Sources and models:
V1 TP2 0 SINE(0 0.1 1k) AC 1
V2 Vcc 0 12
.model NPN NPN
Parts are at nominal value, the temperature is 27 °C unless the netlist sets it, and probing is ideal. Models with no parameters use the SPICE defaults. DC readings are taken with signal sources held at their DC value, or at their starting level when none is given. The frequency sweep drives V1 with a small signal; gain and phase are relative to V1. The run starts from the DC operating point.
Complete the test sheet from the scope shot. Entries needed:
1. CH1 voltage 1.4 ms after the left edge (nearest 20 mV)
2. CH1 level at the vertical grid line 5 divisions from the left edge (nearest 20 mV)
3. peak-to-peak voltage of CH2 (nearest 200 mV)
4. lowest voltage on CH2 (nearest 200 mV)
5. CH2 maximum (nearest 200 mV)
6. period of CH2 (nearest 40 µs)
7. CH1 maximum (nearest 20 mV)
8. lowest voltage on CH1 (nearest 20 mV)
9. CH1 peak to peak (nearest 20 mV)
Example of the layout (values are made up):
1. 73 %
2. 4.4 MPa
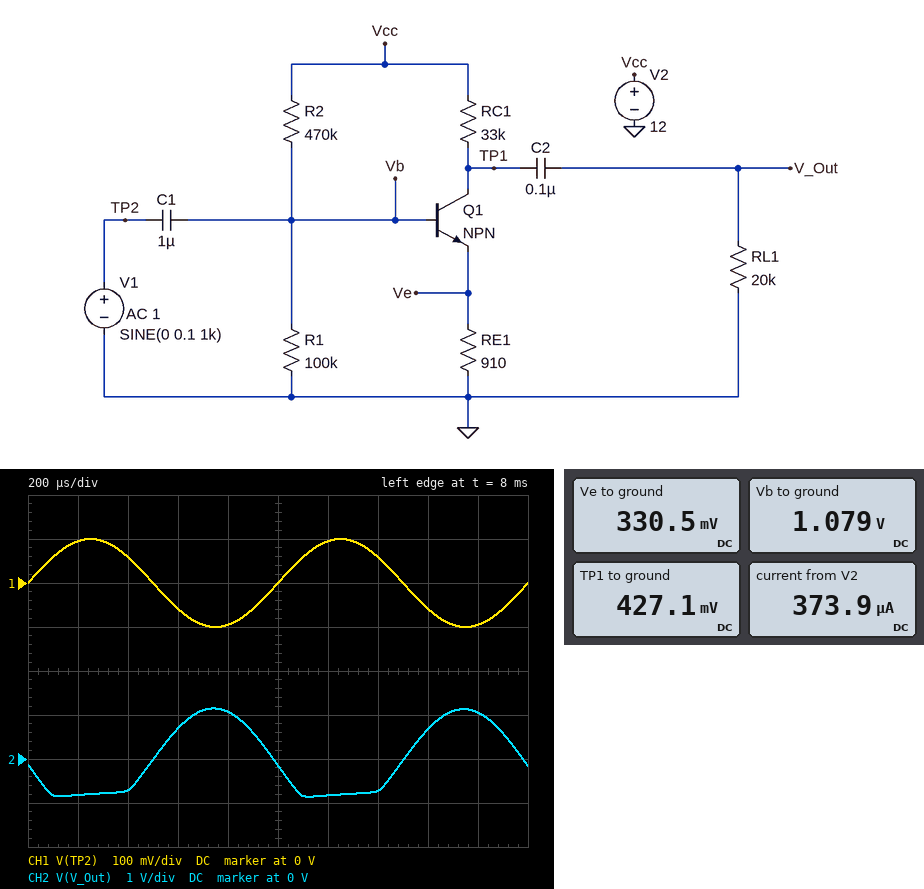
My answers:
1. 60 mV
2. 0 V
3. 2.0 V
4. -800 mV
5. 1.2 V
6. 1.00 ms
7. 100 mV
8. -100 mV
9. 200 mV
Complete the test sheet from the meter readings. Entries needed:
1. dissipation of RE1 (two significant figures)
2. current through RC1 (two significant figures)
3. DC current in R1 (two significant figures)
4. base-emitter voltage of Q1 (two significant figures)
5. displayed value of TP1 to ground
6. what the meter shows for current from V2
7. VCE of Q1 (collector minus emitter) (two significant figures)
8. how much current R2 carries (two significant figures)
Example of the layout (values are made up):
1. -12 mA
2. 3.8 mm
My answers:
1. 120 µW
2. 350 µA
3. 11 µA
4. 750 mV
5. 427.1 mV
6. 373.9 µA
7. 97 mV
8. 23 µA
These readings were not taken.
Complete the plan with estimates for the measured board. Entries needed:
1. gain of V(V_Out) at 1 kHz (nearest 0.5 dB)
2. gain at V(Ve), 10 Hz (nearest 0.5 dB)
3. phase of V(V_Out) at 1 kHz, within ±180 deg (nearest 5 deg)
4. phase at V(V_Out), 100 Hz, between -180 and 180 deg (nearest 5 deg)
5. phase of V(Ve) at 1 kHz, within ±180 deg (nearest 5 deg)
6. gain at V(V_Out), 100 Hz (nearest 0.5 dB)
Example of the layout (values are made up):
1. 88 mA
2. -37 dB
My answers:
1. 3.0 dB
2. -24.5 dB
3. -170 deg
4. -90 deg
5. 10 deg
6. -3.0 dB
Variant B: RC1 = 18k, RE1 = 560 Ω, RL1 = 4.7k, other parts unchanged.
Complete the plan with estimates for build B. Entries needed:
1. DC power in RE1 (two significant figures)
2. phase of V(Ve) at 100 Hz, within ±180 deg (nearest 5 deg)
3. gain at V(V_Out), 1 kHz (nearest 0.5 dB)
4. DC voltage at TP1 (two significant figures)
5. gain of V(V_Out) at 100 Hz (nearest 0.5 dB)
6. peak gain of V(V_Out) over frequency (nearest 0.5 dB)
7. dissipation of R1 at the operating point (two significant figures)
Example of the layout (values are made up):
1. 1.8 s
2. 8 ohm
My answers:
1. 240 µW
2. 70 deg
3. 9.0 dB
4. 490 mV
5. -3.5 dB
6. 9.5 dB
7. 13 µW
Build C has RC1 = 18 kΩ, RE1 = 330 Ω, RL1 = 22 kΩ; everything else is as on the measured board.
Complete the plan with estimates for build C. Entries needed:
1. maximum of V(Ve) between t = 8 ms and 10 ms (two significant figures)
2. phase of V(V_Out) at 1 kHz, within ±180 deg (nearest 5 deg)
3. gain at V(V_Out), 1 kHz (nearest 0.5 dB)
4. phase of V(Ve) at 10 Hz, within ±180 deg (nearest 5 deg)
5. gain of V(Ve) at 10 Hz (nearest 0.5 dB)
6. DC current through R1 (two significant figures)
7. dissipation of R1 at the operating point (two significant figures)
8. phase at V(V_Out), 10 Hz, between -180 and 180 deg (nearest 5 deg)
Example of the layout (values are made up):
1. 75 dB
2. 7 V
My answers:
1. 270 mV
2. -160 deg
3. 15.0 dB
4. 90 deg
5. -32.5 dB
6. 9.8 µA
7. 9.6 µW
8. -10 deg
